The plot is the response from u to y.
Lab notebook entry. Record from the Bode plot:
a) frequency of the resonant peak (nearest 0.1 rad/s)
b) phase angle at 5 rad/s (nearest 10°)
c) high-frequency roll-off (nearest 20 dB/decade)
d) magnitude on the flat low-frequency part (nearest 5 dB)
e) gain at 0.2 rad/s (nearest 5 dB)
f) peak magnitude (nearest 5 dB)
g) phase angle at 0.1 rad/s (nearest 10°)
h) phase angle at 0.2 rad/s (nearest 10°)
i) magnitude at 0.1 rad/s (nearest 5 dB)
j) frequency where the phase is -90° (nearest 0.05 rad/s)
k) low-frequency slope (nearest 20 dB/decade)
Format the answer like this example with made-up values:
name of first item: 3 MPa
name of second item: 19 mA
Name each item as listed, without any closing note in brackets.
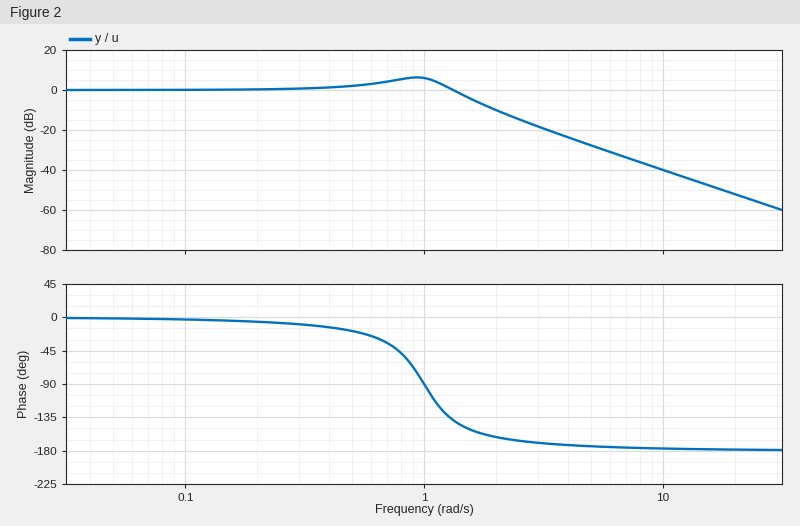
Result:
frequency of the resonant peak: 0.9 rad/s
phase angle at 5 rad/s: -170°
high-frequency roll-off: -40 dB/decade
magnitude on the flat low-frequency part: 0 dB
gain at 0.2 rad/s: 0 dB
peak magnitude: 5 dB
phase angle at 0.1 rad/s: 0°
phase angle at 0.2 rad/s: -10°
magnitude at 0.1 rad/s: 0 dB
frequency where the phase is -90°: 1.00 rad/s
low-frequency slope: 0 dB/decade
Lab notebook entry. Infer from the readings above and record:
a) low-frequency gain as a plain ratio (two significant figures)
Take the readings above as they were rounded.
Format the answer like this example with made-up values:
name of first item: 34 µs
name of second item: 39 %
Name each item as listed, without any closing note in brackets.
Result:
low-frequency gain as a plain ratio: 1.0
